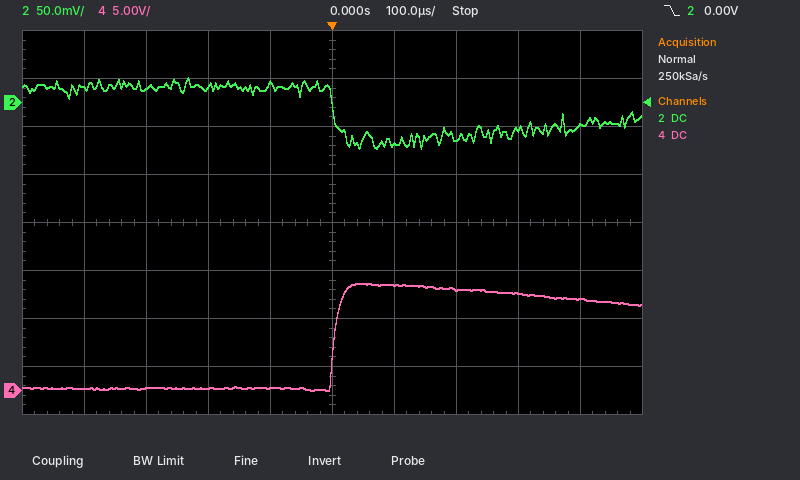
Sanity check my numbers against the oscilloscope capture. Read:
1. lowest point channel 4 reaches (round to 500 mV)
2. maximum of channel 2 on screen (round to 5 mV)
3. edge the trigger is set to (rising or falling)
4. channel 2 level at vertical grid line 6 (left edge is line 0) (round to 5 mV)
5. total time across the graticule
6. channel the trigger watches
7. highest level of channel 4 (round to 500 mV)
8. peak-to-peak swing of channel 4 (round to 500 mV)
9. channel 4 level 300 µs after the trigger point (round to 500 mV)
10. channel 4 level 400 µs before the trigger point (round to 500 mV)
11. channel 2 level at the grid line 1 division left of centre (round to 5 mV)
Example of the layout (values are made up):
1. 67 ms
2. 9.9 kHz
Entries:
1. 0.0 V
2. 25 mV
3. falling
4. -45 mV
5. 1 ms
6. channel 2
7. 11.0 V
8. 11.0 V
9. 10.0 V
10. 0.0 V
11. 20 mV
